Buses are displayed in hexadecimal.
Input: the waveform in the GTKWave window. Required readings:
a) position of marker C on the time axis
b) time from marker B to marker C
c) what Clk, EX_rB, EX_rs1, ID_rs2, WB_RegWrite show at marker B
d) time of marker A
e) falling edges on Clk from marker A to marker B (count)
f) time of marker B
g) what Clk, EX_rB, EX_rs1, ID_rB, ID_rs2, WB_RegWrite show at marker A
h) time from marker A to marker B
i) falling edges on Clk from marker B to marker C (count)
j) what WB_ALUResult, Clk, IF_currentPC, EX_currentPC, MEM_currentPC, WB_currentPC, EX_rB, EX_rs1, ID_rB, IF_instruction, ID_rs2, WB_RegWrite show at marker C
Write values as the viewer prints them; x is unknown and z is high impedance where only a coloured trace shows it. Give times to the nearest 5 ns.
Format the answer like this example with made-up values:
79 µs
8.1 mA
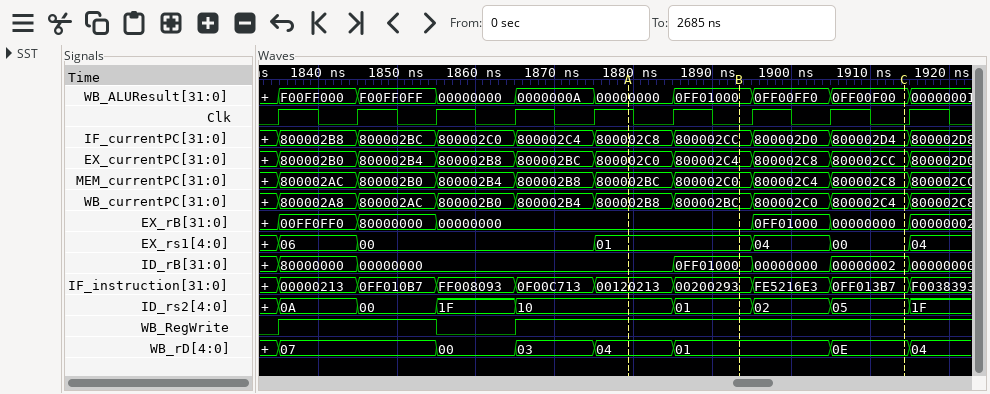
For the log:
1915 ns
20 ns
Clk=0, EX_rB=00000000, EX_rs1=01, ID_rs2=01, WB_RegWrite=1
1880 ns
2
1895 ns
Clk=1, EX_rB=00000000, EX_rs1=01, ID_rB=00000000, ID_rs2=10, WB_RegWrite=1
15 ns
2
WB_ALUResult=0FF00F00, Clk=0, IF_currentPC=800002D4, EX_currentPC=800002CC, MEM_currentPC=800002C8, WB_currentPC=800002C4, EX_rB=00000000, EX_rs1=00, ID_rB=00000002, IF_instruction=0FF013B7, ID_rs2=05, WB_RegWrite=1
